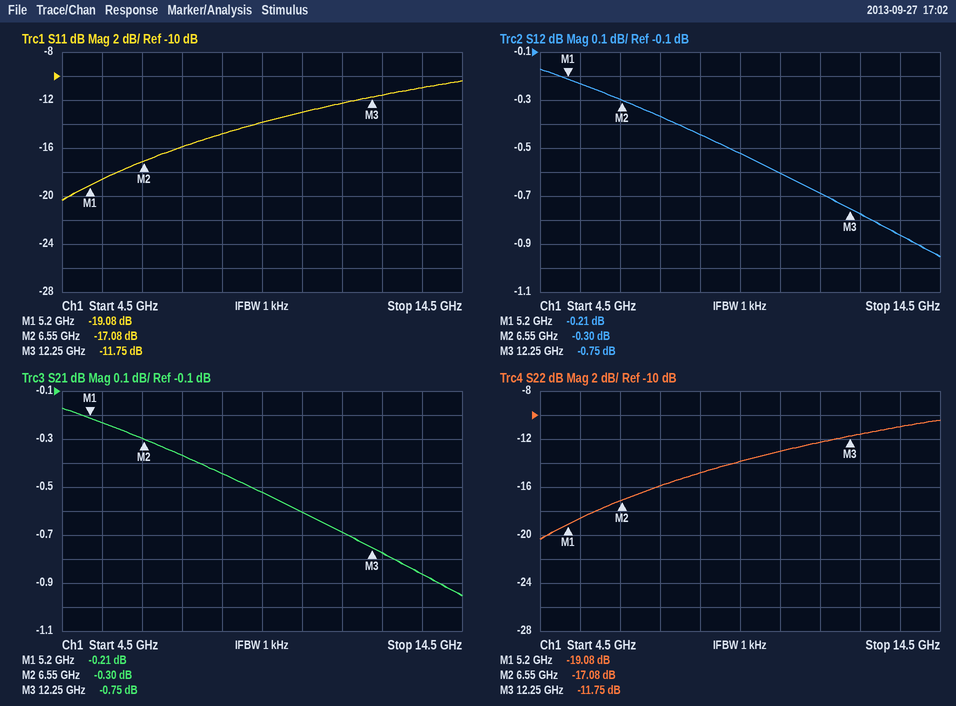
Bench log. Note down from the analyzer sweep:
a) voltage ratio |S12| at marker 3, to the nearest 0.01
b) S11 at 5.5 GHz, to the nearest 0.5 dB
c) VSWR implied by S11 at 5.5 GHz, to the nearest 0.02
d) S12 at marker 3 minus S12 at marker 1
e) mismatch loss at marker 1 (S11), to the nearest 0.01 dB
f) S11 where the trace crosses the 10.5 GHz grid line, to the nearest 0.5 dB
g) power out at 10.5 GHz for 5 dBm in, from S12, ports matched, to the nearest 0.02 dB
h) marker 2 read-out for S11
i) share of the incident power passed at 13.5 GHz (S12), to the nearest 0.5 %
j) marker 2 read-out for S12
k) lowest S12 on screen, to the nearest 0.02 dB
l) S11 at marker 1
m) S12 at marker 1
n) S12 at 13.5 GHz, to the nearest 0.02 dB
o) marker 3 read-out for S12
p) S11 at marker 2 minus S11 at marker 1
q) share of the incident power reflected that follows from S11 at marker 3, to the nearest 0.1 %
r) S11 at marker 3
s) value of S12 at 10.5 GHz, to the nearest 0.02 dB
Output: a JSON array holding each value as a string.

["0.92", "-18.5 dB", "1.26", "-0.54 dB", "0.05 dB", "-13.0 dB", "4.40 dBm", "-17.08 dB", "82.0 %", "-0.30 dB", "-0.96 dB", "-19.08 dB", "-0.21 dB", "-0.86 dB", "-0.75 dB", "2.00 dB", "6.7 %", "-11.75 dB", "-0.60 dB"]
